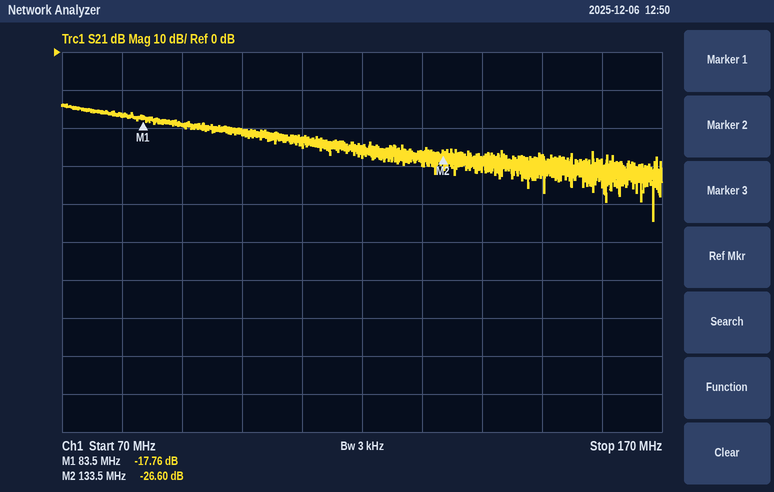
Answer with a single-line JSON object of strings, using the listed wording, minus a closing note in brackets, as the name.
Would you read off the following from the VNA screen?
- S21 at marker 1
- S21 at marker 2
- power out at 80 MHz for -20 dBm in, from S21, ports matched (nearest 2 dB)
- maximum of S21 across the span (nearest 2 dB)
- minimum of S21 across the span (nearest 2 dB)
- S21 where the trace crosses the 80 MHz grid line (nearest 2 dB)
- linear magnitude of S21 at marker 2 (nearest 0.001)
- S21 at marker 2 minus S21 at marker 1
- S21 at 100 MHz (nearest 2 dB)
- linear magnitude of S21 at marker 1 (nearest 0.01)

{"S21 at marker 1": "-17.76 dB", "S21 at marker 2": "-26.60 dB", "power out at 80 MHz for -20 dBm in, from S21, ports matched": "-36 dBm", "maximum of S21 across the span": "-14 dB", "minimum of S21 across the span": "-44 dB", "S21 where the trace crosses the 80 MHz grid line": "-16 dB", "linear magnitude of S21 at marker 2": "0.047", "S21 at marker 2 minus S21 at marker 1": "-8.84 dB", "S21 at 100 MHz": "-22 dB", "linear magnitude of S21 at marker 1": "0.13"}
